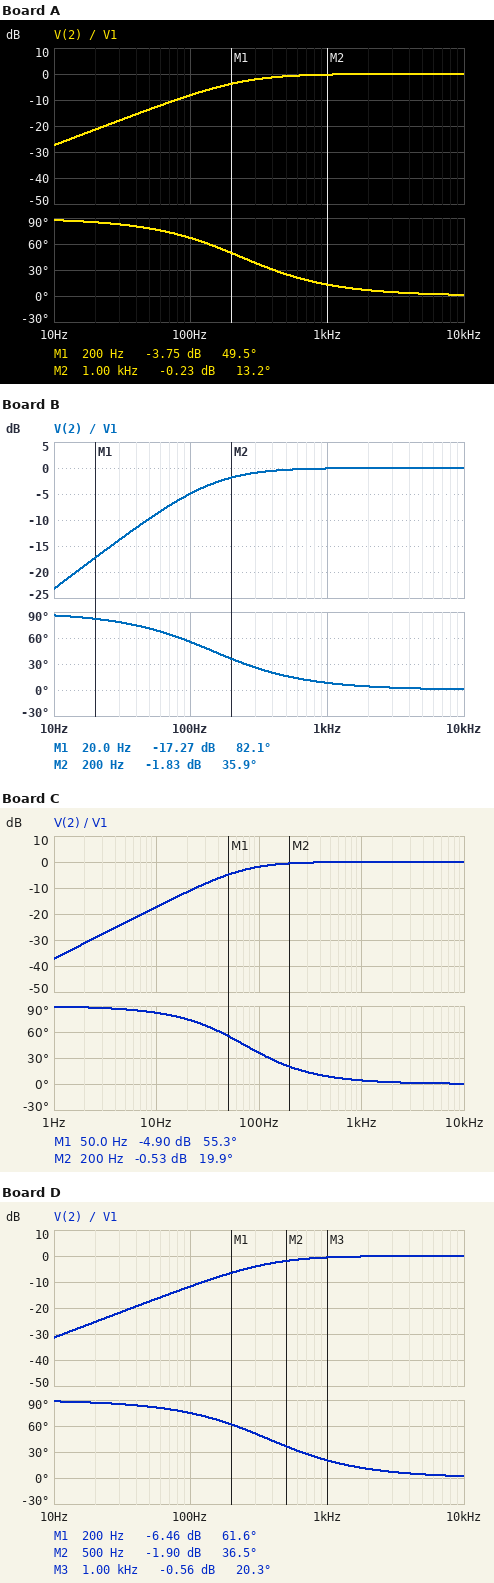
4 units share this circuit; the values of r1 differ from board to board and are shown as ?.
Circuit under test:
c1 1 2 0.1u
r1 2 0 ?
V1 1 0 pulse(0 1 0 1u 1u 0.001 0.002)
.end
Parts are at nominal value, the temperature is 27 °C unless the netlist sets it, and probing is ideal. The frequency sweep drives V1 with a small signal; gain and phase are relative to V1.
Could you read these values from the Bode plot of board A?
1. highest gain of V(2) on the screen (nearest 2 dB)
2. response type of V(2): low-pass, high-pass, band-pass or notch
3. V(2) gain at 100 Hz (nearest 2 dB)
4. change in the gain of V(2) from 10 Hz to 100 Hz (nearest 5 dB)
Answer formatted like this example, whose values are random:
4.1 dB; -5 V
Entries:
0 dB; high-pass; -8 dB; 20 dB
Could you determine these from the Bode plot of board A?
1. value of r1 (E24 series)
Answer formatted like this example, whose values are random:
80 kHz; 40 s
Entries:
6.8 kΩ
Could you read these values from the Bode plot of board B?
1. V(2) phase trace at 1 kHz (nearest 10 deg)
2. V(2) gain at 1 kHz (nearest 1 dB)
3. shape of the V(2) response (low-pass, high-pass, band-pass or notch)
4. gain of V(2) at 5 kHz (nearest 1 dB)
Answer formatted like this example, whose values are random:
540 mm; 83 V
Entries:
10 deg; 0 dB; high-pass; 0 dB
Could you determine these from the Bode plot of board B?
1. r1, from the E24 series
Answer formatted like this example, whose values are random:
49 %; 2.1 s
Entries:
11 kΩ
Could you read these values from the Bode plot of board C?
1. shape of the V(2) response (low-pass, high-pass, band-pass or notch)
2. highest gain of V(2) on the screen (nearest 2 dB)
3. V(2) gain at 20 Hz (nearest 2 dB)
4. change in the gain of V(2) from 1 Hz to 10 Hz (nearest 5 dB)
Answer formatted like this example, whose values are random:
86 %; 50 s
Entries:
high-pass; 0 dB; -12 dB; 20 dB
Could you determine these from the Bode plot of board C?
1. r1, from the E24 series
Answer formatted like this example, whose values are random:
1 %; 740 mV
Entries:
22 kΩ
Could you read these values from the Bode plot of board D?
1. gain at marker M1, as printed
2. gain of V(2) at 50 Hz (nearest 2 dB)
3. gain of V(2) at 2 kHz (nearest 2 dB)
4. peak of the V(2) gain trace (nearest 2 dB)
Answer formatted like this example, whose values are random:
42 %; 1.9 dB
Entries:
-6.46 dB; -18 dB; 0 dB; 0 dB
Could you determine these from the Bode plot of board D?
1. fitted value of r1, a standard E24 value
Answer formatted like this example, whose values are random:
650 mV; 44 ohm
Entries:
4.3 kΩ
